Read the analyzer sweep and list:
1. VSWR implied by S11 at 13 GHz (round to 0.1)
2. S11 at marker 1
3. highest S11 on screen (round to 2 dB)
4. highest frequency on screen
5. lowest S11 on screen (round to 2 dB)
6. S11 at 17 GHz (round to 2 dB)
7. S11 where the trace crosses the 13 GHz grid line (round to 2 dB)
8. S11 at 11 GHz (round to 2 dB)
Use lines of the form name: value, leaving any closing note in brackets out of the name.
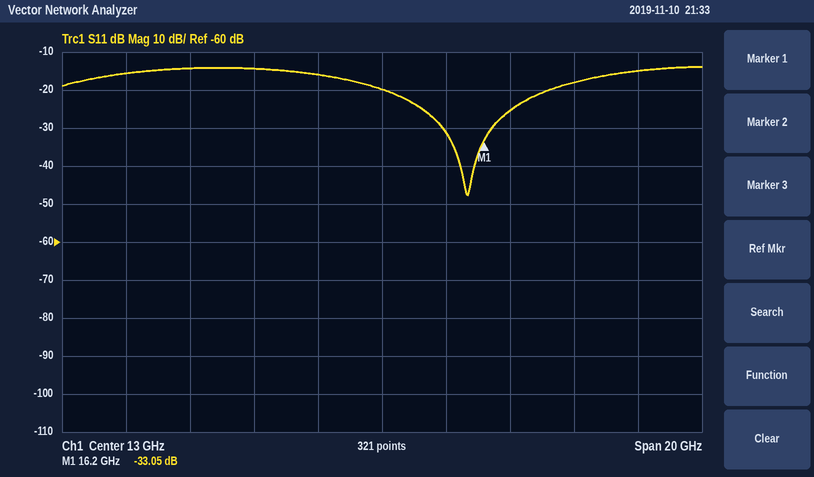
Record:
VSWR implied by S11 at 13 GHz: 1.2
S11 at marker 1: -33.05 dB
highest S11 on screen: -14 dB
highest frequency on screen: 23 GHz
lowest S11 on screen: -48 dB
S11 at 17 GHz: -26 dB
S11 where the trace crosses the 13 GHz grid line: -20 dB
S11 at 11 GHz: -16 dB
